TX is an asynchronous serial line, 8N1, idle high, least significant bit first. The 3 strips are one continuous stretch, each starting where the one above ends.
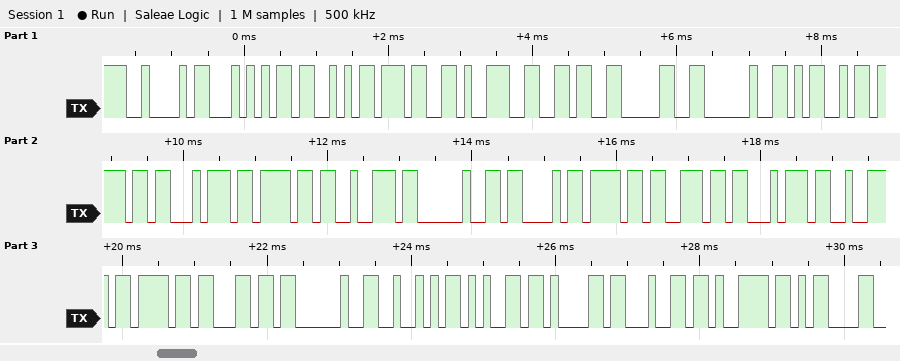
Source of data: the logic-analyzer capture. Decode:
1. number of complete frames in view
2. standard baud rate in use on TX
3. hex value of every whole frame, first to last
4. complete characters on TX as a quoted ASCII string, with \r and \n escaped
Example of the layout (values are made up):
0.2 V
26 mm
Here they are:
28
9600 baud
42 54 53 37 39 36 30 20 4D 6F 74 6F 72 20 43 6F 6E 74 72 6F 6C 20 52 65 61 64 79 0D
"BTS7960 Motor Control Ready\r"
